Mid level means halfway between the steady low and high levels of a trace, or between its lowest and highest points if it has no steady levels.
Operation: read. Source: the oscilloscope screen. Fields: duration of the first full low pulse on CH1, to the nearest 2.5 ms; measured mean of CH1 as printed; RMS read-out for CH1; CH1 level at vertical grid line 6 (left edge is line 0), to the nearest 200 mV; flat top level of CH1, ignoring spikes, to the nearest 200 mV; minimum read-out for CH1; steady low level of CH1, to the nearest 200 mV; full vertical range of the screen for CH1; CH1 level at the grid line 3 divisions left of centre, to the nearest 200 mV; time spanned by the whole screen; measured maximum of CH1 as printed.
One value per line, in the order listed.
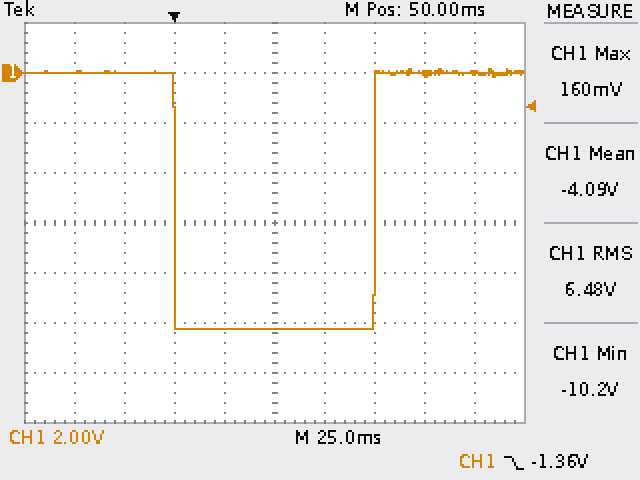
100.0 ms
-4.09 V
6.48 V
-10.2 V
0.0 V
-10.2 V
-10.2 V
16 V
0.0 V
250 ms
160 mV
